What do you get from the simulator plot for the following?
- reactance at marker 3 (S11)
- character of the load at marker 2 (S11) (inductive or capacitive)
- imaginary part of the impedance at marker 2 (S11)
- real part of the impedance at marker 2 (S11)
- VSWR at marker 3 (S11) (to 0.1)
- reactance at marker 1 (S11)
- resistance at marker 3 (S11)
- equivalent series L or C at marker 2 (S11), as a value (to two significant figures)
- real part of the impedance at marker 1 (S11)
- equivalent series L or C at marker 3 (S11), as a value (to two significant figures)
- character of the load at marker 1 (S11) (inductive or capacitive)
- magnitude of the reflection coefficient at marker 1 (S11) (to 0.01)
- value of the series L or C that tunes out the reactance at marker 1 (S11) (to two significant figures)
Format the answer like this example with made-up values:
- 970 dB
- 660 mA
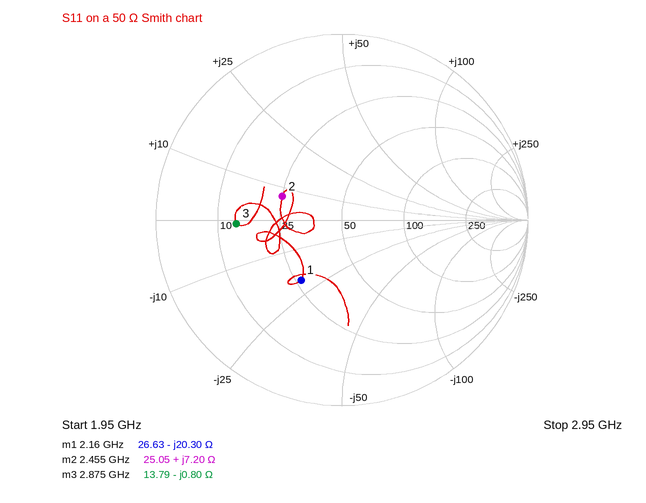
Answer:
- -0.80 Ω
- inductive
- +7.20 Ω
- 25.05 Ω
- 3.6
- -20.30 Ω
- 13.79 Ω
- 470 pH
- 26.63 Ω
- 69 pF
- capacitive
- 0.39
- 1.5 nH
